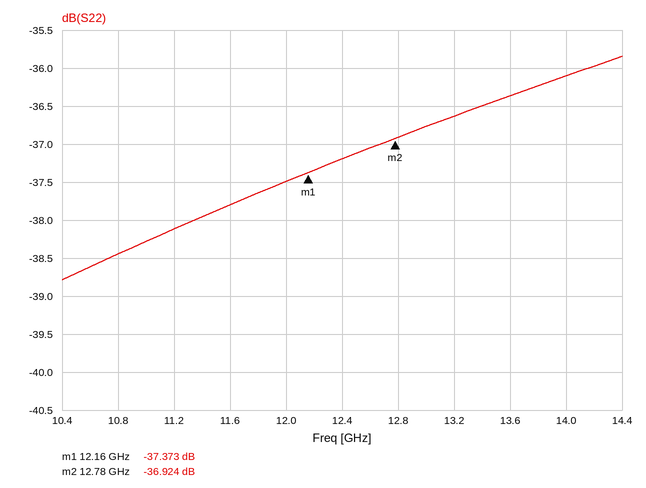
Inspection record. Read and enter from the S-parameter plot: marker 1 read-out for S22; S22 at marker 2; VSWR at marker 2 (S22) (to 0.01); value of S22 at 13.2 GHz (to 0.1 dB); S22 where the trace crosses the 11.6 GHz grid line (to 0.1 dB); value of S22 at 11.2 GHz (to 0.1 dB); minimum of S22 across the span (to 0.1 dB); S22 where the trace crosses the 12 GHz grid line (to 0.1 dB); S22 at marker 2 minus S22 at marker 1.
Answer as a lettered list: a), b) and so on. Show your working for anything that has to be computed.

a) -37.373 dB
b) -36.924 dB
c) (1 + 0.0142)/(1 − 0.0142) ≈ 1.03
d) -36.6 dB
e) -37.8 dB
f) -38.1 dB
g) -38.8 dB
h) -37.5 dB
i) -36.924 − (-37.373) = 0.449 dB
